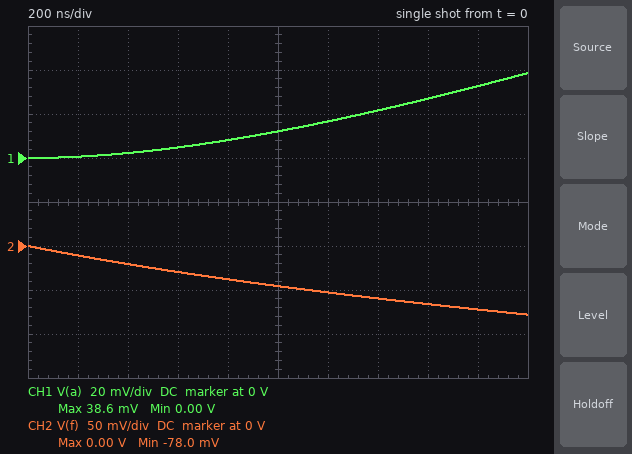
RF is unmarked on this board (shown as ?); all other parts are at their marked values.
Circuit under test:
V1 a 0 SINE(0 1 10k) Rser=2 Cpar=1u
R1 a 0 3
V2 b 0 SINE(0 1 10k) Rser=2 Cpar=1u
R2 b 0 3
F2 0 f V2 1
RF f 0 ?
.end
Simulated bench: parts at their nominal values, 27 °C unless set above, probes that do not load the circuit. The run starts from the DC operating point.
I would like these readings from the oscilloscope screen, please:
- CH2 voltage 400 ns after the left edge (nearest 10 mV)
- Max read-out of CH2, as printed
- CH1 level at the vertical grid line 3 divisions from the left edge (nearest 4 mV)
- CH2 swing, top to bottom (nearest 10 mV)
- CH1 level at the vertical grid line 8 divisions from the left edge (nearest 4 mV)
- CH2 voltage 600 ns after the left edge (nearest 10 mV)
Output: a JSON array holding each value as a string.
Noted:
["-20 mV", "0.00 V", "4 mV", "80 mV", "28 mV", "-30 mV"]
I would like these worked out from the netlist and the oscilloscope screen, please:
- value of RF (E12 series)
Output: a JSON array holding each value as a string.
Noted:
["1.8 Ω"]
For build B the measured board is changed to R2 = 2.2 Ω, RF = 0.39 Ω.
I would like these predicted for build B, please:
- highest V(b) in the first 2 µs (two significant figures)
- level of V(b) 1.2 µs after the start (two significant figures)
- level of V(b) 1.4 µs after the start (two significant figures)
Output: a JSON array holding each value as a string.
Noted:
["36 mV", "16 mV", "21 mV"]
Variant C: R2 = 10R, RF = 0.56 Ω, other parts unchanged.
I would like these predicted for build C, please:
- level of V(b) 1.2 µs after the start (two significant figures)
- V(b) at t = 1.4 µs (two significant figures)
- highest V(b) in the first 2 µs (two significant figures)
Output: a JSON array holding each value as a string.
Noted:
["18 mV", "24 mV", "44 mV"]
